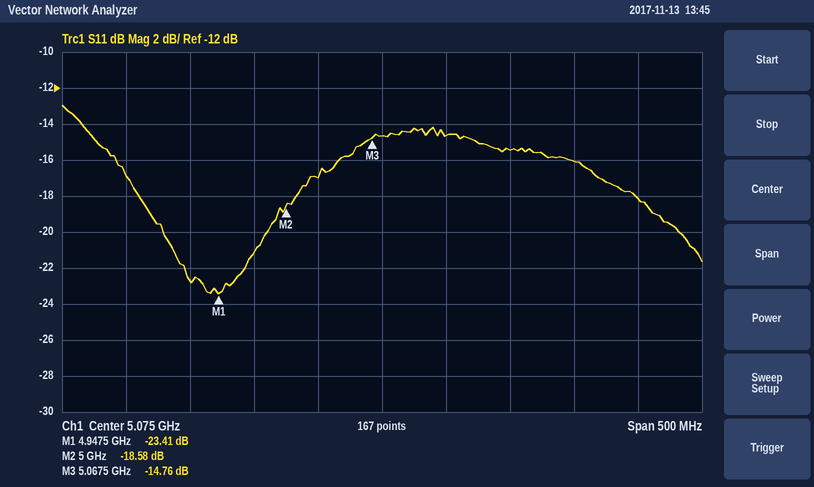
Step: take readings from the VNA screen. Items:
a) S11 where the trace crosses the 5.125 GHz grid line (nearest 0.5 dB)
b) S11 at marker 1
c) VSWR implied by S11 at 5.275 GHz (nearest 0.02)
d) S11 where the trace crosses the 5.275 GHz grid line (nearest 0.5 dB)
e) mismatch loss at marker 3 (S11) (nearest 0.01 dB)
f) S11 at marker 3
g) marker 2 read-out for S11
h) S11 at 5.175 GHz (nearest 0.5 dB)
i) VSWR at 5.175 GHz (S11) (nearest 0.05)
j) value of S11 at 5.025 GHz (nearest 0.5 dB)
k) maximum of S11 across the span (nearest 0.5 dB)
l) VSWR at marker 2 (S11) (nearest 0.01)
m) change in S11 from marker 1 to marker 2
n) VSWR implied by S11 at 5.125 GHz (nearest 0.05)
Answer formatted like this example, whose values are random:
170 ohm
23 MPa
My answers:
-14.5 dB
-23.41 dB
1.28
-18.0 dB
0.15 dB
-14.76 dB
-18.58 dB
-15.5 dB
1.40
-17.0 dB
-13.0 dB
1.27
4.83 dB
1.45
